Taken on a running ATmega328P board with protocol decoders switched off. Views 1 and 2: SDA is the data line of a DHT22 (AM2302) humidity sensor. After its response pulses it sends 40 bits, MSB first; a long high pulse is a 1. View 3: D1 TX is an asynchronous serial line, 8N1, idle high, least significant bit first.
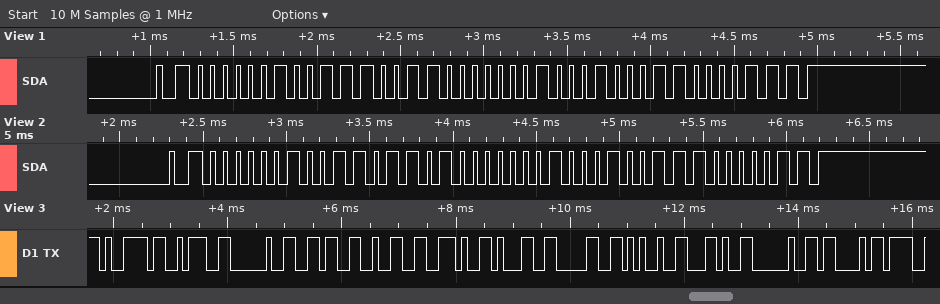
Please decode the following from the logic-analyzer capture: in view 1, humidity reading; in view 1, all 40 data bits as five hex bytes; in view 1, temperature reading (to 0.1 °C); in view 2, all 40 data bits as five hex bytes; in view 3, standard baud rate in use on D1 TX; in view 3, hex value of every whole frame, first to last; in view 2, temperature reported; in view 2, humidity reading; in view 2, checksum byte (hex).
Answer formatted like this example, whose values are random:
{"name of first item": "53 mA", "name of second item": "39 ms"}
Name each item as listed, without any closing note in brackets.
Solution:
{"in view 1, humidity reading": "62.7 %", "in view 1, all 40 data bits as five hex bytes": "02 73 01 11 87", "in view 1, temperature reading": "27.3 °C", "in view 2, all 40 data bits as five hex bytes": "02 6D 01 13 83", "in view 3, standard baud rate in use on D1 TX": "9600 baud", "in view 3, hex value of every whole frame, first to last": "79 3A 20 36 32 2E 31 30 25 2C 20 43", "in view 2, temperature reported": "27.5 °C", "in view 2, humidity reading": "62.1 %", "in view 2, checksum byte": "0x83"}
